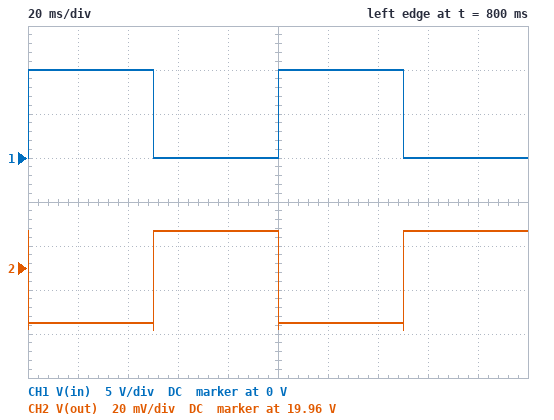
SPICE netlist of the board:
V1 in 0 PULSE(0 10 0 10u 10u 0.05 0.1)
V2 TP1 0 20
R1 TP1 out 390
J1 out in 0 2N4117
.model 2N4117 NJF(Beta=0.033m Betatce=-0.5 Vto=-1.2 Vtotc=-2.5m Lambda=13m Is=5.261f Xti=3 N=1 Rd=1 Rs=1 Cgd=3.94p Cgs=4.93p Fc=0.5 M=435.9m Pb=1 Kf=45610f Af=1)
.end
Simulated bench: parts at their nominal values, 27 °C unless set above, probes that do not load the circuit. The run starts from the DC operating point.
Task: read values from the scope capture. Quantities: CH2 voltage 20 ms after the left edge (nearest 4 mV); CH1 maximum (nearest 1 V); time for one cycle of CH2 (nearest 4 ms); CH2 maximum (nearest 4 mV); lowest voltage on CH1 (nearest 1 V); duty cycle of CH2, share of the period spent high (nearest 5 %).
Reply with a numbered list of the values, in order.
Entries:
1. 19.936 V
2. 10 V
3. 100 ms
4. 19.976 V
5. 0 V
6. 50 %
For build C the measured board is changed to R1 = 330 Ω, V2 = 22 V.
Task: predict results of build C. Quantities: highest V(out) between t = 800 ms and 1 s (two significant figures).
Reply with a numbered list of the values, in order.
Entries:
1. 22 V
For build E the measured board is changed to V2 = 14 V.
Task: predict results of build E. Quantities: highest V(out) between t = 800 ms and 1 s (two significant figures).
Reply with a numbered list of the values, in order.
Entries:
1. 14 V
